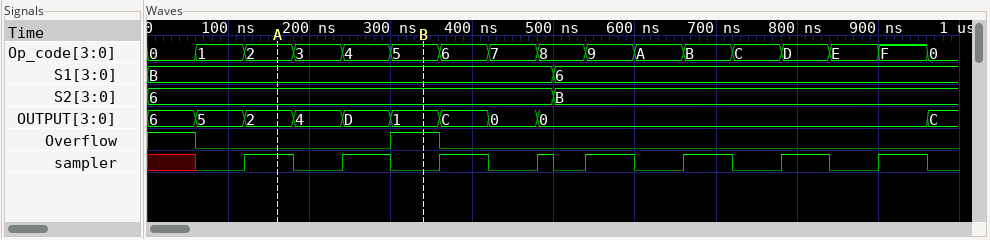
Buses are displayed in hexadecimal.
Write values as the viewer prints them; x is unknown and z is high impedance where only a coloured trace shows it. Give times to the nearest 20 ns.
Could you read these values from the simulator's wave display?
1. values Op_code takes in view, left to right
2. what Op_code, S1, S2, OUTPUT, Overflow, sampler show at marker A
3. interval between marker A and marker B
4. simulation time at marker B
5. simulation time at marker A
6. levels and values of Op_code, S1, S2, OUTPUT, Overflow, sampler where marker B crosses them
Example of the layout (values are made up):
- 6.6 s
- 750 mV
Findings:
- 0, 1, 2, 3, 4, 5, 6, 7, 8, 9, A, B, C, D, E, F, 0
- Op_code=2, S1=B, S2=6, OUTPUT=2, Overflow=0, sampler=1
- 180 ns
- 340 ns
- 160 ns
- Op_code=5, S1=B, S2=6, OUTPUT=1, Overflow=1, sampler=0
